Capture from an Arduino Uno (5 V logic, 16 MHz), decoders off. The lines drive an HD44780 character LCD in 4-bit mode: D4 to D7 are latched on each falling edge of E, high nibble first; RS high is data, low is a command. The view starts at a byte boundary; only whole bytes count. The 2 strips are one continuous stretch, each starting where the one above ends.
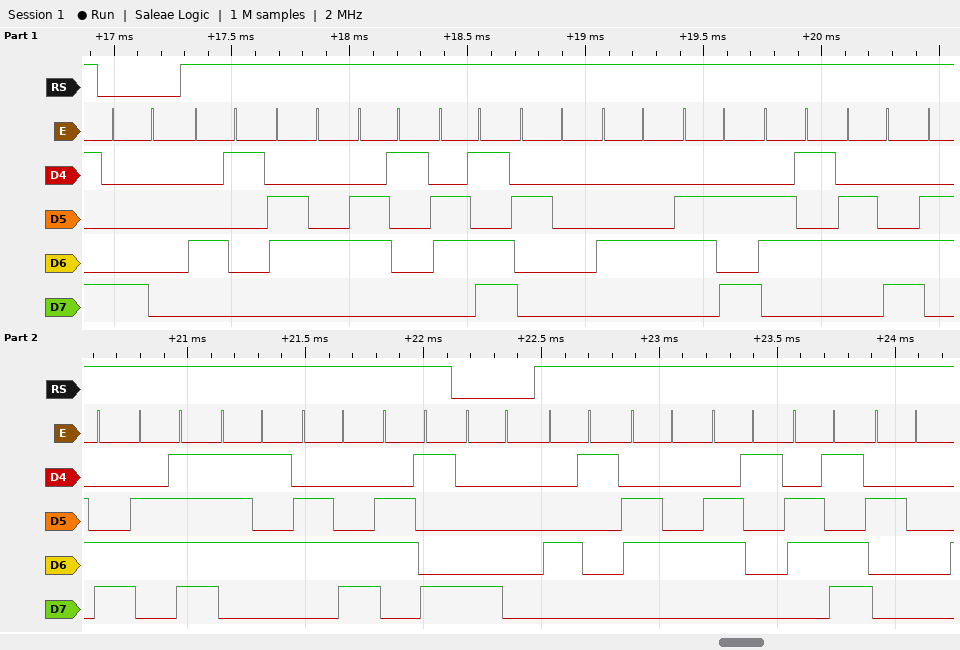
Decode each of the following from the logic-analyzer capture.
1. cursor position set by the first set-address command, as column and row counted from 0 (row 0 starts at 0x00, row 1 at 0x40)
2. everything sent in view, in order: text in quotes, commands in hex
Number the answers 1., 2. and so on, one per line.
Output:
1. column 0, row 0
2. 0x80 "Adam Djellouli" 0x80 "Adam "
